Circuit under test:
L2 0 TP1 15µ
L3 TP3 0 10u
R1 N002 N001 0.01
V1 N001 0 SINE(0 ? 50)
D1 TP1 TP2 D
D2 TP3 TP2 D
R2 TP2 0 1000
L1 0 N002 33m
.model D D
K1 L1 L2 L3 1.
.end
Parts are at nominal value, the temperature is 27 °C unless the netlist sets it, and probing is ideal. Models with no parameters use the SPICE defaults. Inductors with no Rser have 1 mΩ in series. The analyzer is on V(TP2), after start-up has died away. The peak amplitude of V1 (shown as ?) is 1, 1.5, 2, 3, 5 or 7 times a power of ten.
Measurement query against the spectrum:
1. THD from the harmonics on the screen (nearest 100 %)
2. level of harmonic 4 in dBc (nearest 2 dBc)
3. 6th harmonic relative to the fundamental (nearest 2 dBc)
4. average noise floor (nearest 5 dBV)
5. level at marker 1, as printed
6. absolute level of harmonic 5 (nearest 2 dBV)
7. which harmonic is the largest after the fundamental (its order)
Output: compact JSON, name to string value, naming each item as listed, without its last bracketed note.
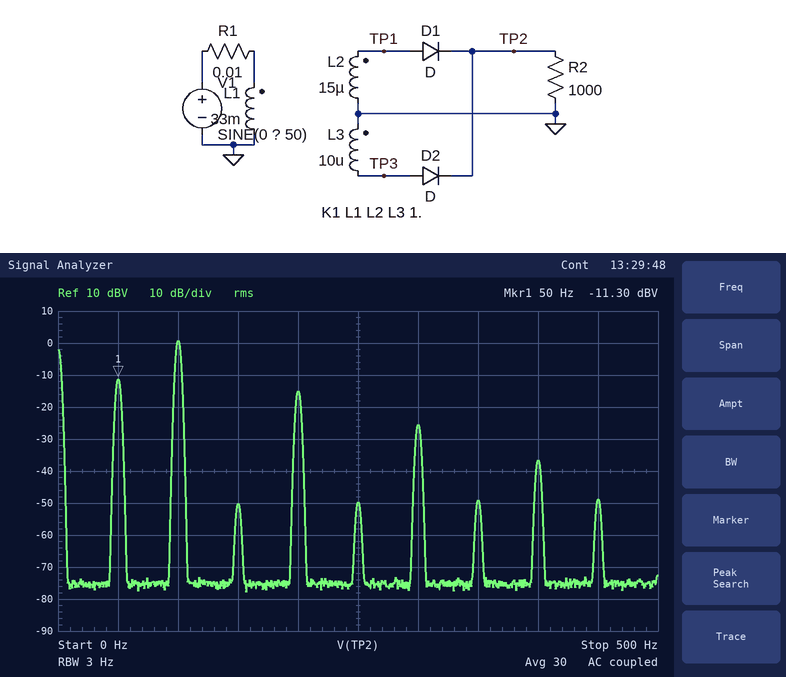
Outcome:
{"THD from the harmonics on the screen": "400 %", "level of harmonic 4 in dBc": "-4 dBc", "6th harmonic relative to the fundamental": "-14 dBc", "average noise floor": "-75 dBV", "level at marker 1, as printed": "-11.30 dBV", "absolute level of harmonic 5": "-50 dBV", "which harmonic is the largest after the fundamental": "2"}
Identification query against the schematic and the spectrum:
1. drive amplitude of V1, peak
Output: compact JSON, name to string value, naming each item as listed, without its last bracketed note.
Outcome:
{"drive amplitude of V1, peak": "200 V"}
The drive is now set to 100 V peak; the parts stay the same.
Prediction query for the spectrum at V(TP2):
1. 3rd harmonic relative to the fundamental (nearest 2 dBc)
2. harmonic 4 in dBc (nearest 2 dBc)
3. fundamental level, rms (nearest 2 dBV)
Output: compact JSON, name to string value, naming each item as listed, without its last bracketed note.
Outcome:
{"3rd harmonic relative to the fundamental": "-26 dBc", "harmonic 4 in dBc": "-12 dBc", "fundamental level, rms": "-18 dBV"}
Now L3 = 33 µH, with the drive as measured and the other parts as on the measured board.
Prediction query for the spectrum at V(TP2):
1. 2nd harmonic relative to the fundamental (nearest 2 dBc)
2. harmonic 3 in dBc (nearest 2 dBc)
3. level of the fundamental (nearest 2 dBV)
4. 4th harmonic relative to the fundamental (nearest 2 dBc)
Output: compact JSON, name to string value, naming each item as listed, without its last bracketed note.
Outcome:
{"2nd harmonic relative to the fundamental": "6 dBc", "harmonic 3 in dBc": "-46 dBc", "level of the fundamental": "-2 dBV", "4th harmonic relative to the fundamental": "-8 dBc"}
